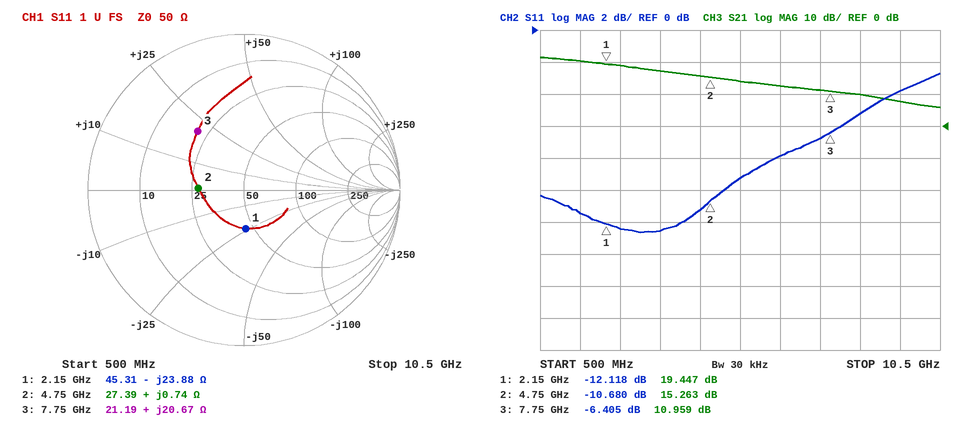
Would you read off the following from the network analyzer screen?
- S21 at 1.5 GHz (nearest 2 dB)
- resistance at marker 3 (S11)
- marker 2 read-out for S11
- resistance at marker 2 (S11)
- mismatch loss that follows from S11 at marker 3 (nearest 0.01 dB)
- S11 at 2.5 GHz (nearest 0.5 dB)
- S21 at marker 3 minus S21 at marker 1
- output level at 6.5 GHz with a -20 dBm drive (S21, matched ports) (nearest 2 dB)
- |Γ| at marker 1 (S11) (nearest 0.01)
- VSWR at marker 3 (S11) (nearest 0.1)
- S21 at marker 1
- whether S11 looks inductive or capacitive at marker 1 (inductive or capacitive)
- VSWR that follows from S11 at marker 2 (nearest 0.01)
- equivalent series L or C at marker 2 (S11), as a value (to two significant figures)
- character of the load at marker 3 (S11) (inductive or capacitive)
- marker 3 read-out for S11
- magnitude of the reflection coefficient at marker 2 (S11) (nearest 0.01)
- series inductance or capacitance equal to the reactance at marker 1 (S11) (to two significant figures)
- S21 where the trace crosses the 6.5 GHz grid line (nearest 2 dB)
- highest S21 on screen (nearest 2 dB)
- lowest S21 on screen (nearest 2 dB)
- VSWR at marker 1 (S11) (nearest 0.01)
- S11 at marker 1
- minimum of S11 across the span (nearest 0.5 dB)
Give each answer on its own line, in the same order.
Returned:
20 dB
21.19 Ω
-10.680 dB
27.39 Ω
1.13 dB
-12.5 dB
-8.488 dB
-8 dBm
0.25
2.8
19.447 dB
capacitive
1.83
25 pH
inductive
-6.405 dB
0.29
3.1 pF
12 dB
22 dB
6 dB
1.66
-12.118 dB
-12.5 dB
